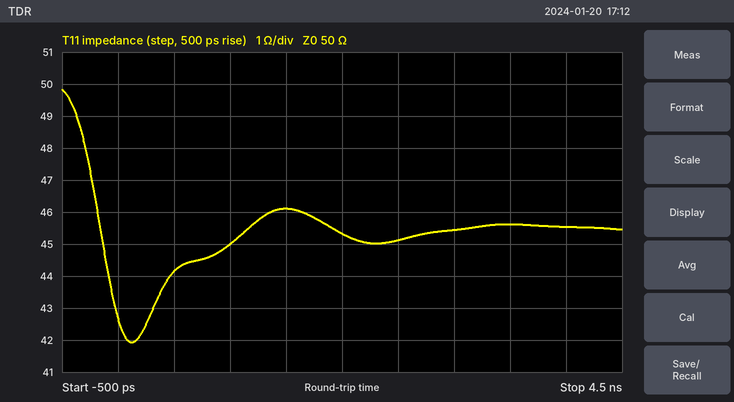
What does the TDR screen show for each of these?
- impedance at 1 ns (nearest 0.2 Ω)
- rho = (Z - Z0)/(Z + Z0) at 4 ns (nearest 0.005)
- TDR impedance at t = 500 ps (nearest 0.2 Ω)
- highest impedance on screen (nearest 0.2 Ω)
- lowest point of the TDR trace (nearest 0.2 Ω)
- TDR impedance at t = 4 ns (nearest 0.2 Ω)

45.0 Ω
-0.045
44.2 Ω
49.8 Ω
42.0 Ω
45.6 Ω
